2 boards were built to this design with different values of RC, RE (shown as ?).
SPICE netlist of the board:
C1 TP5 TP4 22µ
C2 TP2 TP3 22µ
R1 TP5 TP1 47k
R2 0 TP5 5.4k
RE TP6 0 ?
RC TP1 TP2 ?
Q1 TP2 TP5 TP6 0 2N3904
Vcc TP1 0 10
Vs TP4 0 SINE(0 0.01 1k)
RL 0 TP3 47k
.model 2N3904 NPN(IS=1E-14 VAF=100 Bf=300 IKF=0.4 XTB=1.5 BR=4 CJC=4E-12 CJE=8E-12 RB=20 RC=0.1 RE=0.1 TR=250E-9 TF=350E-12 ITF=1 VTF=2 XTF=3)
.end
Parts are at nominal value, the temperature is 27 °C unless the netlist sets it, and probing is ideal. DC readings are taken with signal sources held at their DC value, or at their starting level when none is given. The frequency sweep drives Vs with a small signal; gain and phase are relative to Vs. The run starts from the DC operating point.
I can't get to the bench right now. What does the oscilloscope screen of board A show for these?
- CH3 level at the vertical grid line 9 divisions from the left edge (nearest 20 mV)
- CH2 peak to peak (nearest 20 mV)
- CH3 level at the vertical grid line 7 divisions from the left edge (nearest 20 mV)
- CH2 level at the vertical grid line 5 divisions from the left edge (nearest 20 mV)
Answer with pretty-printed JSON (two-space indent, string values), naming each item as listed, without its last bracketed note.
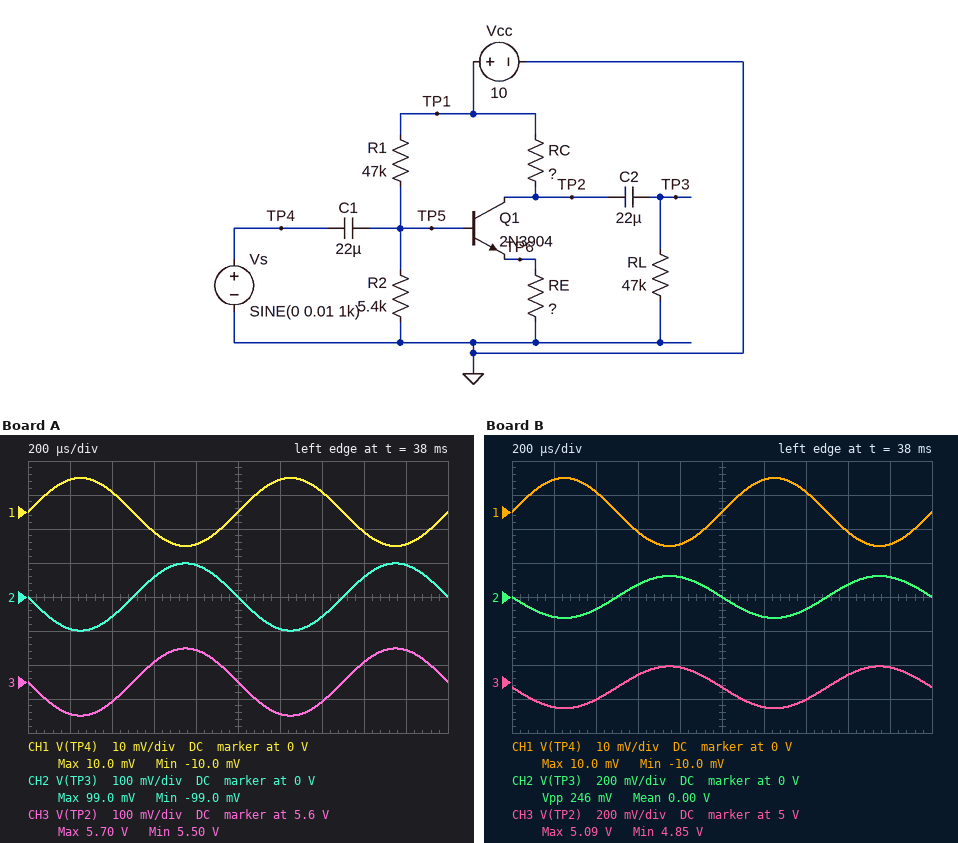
{
  "CH3 level at the vertical grid line 9 divisions from the left edge": "5.70 V",
  "CH2 peak to peak": "200 mV",
  "CH3 level at the vertical grid line 7 divisions from the left edge": "5.54 V",
  "CH2 level at the vertical grid line 5 divisions from the left edge": "0 V"
}
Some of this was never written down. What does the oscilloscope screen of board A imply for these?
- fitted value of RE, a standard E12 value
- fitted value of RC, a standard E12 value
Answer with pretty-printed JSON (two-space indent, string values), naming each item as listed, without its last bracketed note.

{
  "fitted value of RE, a standard E12 value": "470 Ω",
  "fitted value of RC, a standard E12 value": "5.6 kΩ"
}
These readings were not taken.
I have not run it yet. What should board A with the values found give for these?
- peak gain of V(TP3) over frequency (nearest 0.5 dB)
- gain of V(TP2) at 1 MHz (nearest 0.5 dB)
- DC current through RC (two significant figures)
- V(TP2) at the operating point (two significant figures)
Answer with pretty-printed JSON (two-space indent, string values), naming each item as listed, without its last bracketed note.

{
  "peak gain of V(TP3) over frequency": "20.0 dB",
  "gain of V(TP2) at 1 MHz": "20.0 dB",
  "DC current through RC": "790 µA",
  "V(TP2) at the operating point": "5.6 V"
}
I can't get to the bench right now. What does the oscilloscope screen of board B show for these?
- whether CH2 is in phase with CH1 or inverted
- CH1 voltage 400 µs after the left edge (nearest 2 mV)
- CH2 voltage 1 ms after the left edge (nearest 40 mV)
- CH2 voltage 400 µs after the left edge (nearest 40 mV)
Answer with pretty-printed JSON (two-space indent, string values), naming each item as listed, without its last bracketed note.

{
  "whether CH2 is in phase with CH1 or inverted": "inverted",
  "CH1 voltage 400 µs after the left edge": "6 mV",
  "CH2 voltage 1 ms after the left edge": "0 V",
  "CH2 voltage 400 µs after the left edge": "-80 mV"
}
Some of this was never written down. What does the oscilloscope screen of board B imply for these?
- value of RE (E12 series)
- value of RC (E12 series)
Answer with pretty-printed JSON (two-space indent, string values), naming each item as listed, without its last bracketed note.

{
  "value of RE": "270 Ω",
  "value of RC": "3.9 kΩ"
}
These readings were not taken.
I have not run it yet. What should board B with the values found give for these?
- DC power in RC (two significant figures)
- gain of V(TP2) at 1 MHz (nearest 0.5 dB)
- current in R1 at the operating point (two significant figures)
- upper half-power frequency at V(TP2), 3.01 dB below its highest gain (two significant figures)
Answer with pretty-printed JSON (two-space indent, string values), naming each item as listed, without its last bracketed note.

{
  "DC power in RC": "6.5 mW",
  "gain of V(TP2) at 1 MHz": "22.0 dB",
  "current in R1 at the operating point": "190 µA",
  "upper half-power frequency at V(TP2), 3.01 dB below its highest gain": "19 MHz"
}
